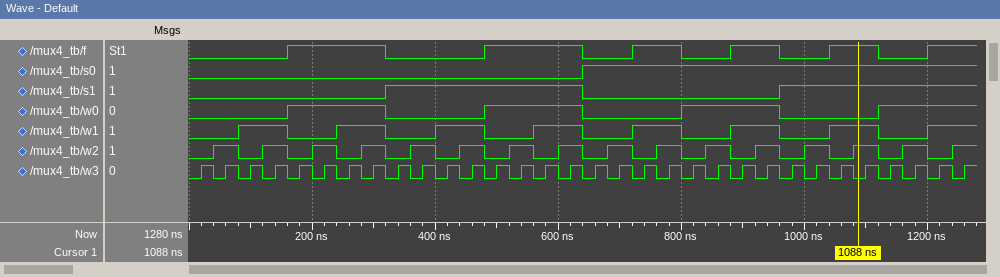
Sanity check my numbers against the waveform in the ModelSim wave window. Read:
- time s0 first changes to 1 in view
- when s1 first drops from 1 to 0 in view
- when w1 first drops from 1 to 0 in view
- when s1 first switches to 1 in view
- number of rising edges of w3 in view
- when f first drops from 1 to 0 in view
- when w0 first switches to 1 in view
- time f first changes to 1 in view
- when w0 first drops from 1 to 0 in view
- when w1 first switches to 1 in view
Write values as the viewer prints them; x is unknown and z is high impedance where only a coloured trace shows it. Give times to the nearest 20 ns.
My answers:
640 ns
640 ns
160 ns
320 ns
32
320 ns
160 ns
160 ns
320 ns
80 ns
